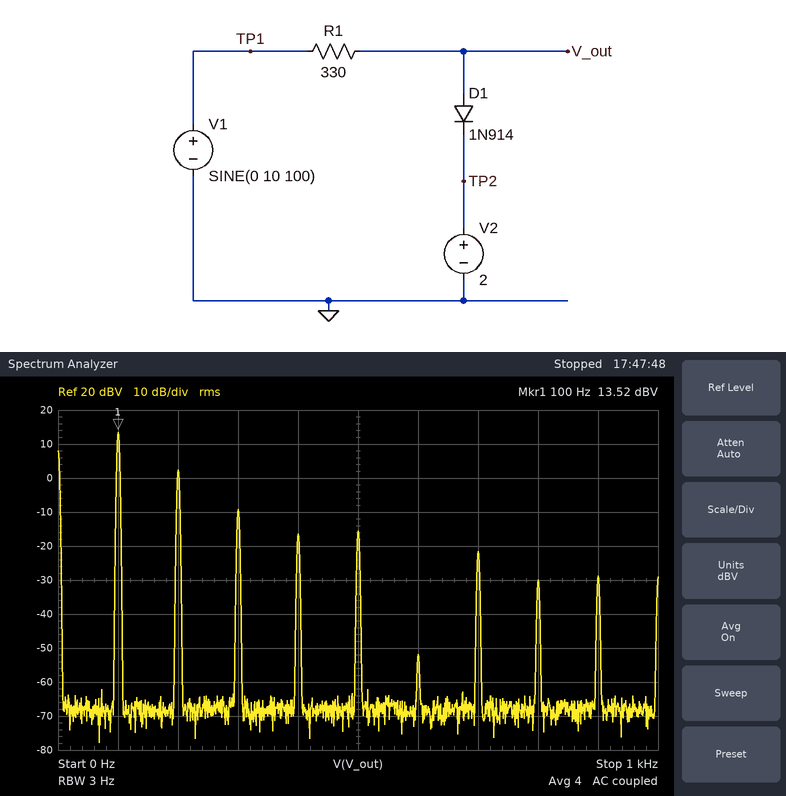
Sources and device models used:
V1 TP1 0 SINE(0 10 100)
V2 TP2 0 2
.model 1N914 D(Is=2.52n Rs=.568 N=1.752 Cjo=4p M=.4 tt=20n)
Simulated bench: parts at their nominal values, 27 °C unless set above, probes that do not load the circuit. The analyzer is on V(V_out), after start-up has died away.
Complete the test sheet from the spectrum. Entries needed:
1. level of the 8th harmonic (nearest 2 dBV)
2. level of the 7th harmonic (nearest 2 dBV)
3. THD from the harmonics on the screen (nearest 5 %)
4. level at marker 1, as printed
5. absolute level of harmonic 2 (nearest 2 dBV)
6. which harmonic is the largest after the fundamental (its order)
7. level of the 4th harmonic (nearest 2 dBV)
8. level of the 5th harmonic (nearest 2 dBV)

-30 dBV
-22 dBV
30 %
13.52 dBV
2 dBV
2
-16 dBV
-16 dBV
